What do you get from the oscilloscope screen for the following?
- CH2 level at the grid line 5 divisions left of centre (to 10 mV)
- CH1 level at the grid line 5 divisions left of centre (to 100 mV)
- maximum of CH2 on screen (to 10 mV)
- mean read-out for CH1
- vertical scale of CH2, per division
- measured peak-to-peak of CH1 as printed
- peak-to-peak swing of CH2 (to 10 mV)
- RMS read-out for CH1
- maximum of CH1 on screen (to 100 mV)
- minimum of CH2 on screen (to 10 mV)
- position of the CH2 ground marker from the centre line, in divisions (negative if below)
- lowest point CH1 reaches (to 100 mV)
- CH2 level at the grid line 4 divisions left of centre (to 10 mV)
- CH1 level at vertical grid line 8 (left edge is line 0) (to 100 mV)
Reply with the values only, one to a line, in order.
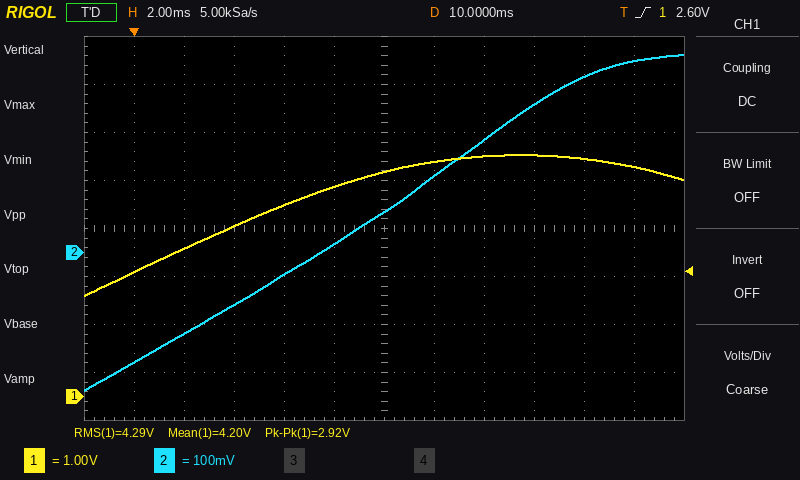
-230 mV
2.6 V
410 mV
4.20 V
100 mV
2.92 V
700 mV
4.29 V
5.0 V
-290 mV
-0.5 div
2.1 V
-170 mV
5.0 V
